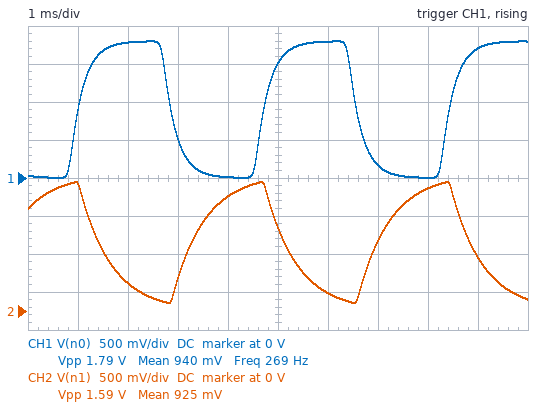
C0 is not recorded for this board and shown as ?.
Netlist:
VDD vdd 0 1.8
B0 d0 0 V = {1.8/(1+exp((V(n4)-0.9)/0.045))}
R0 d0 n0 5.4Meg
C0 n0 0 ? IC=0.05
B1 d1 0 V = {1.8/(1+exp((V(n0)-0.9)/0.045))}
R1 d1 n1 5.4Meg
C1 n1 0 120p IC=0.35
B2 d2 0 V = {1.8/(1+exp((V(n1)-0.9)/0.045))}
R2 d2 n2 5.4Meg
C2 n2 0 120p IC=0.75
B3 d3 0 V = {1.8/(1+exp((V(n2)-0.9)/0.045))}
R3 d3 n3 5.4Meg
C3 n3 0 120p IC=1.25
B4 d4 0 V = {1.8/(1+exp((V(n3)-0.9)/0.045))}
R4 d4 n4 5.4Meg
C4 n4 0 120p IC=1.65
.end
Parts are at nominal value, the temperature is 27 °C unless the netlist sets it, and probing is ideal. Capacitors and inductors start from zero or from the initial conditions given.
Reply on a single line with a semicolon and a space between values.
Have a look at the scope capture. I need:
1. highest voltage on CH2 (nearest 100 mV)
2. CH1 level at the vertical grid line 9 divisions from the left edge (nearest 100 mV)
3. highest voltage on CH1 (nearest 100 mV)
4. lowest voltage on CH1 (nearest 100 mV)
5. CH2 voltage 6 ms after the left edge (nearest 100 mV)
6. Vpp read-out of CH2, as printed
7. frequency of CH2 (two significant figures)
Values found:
1.7 V; 1.7 V; 1.8 V; 0 V; 200 mV; 1.59 V; 270 Hz
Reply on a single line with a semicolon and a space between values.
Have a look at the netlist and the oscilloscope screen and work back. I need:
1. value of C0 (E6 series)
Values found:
47 pF
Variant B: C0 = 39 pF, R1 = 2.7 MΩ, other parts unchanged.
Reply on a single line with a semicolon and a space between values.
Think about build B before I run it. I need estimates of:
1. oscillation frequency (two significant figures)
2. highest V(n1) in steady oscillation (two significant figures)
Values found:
320 Hz; 1.8 V
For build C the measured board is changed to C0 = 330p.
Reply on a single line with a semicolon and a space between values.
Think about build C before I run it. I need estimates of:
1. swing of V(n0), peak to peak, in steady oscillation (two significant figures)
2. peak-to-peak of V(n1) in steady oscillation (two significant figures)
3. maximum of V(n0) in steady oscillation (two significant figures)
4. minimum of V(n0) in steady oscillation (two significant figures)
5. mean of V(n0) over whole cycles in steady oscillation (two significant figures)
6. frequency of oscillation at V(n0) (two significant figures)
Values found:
1.1 V; 1.7 V; 1.5 V; 340 mV; 900 mV; 190 Hz
